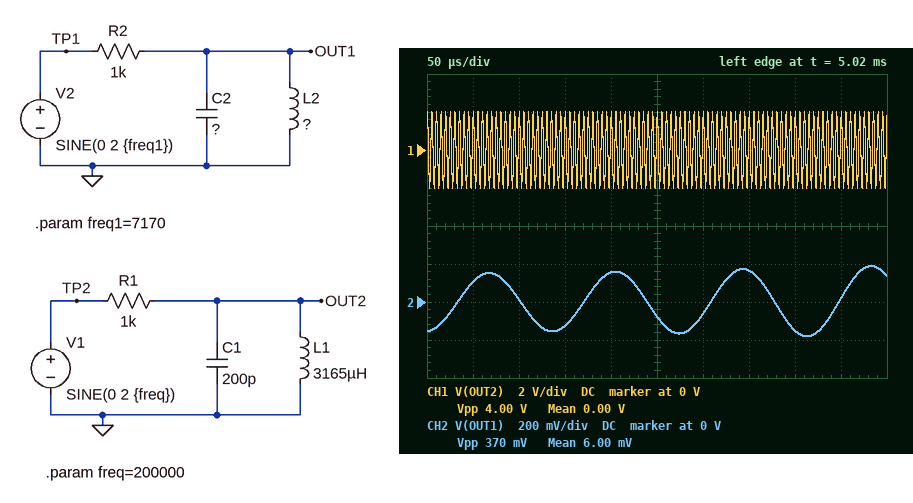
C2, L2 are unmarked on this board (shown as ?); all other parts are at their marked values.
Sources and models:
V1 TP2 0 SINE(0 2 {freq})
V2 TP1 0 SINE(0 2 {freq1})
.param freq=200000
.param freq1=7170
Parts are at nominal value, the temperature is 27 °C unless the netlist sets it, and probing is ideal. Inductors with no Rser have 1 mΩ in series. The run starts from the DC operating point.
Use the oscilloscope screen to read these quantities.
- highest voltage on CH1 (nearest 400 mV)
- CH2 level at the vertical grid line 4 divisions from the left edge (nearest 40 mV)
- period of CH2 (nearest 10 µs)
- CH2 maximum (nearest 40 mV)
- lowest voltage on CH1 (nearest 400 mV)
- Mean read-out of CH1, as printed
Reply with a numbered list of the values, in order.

1. 2.0 V
2. 160 mV
3. 140 µs
4. 200 mV
5. -2.0 V
6. 0.00 V
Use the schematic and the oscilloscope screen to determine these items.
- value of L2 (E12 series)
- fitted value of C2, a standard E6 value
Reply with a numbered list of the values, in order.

1. 390 µH
2. 1.5 µF
